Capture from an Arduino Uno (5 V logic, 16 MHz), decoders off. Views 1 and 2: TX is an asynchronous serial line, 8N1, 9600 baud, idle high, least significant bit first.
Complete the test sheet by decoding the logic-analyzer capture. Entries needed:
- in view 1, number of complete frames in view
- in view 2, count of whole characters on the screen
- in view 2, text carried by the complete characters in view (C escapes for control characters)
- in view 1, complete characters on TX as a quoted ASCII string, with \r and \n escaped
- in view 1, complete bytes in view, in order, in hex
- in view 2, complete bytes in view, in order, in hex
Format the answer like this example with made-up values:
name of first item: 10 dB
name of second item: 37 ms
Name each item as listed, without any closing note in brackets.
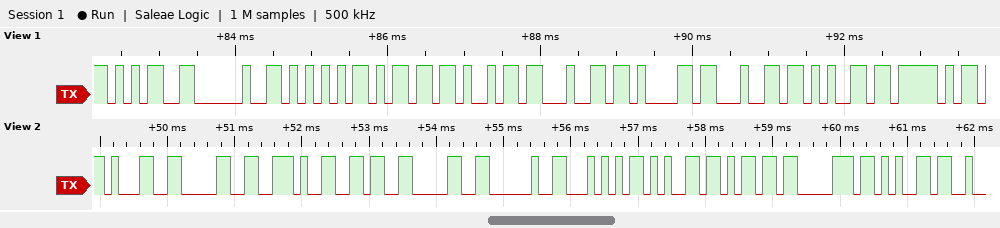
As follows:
in view 1, number of complete frames in view: 10
in view 2, count of whole characters on the screen: 11
in view 2, text carried by the complete characters in view: "10.60 Tempe"
in view 1, complete characters on TX as a quoted ASCII string, with \r and \n escaped: "5 Umidade_"
in view 1, complete bytes in view, in order, in hex: 35 20 55 6D 69 64 61 64 65 5F
in view 2, complete bytes in view, in order, in hex: 31 30 2E 36 30 20 54 65 6D 70 65
